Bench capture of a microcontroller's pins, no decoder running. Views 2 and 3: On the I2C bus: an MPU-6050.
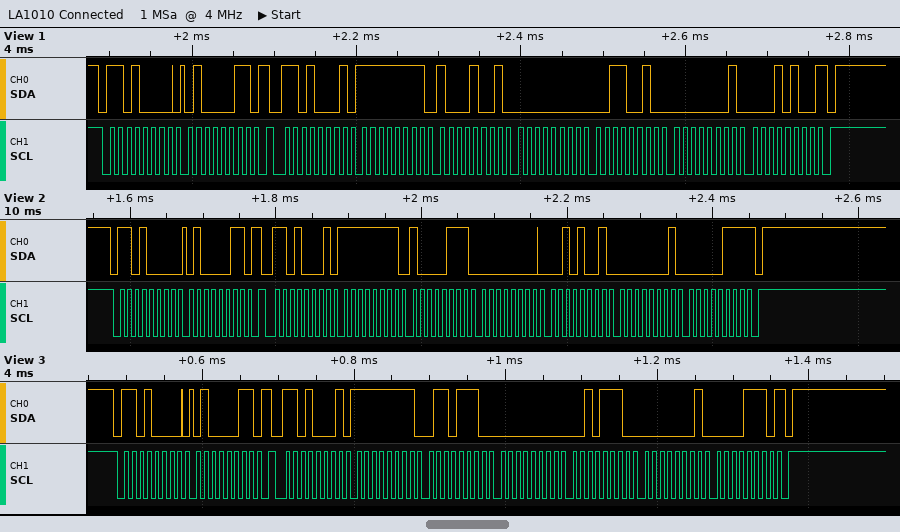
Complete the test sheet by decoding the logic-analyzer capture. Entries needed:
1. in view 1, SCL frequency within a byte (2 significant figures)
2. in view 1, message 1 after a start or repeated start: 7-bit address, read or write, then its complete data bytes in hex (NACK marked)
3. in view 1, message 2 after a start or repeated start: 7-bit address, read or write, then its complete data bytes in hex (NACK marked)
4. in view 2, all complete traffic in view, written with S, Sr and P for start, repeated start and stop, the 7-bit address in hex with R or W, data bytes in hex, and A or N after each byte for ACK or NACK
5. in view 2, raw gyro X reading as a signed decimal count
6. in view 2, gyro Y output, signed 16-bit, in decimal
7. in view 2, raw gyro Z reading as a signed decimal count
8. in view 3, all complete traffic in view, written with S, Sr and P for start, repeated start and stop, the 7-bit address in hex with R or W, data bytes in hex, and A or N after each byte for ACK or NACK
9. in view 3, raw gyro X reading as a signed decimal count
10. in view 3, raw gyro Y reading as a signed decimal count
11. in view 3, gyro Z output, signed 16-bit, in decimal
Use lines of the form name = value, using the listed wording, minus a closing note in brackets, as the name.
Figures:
in view 1, SCL frequency within a byte = 100 kHz
in view 1, message 1 after a start or repeated start: 7-bit address, read or write, then its complete data bytes in hex = 0x68 write: 43
in view 1, message 2 after a start or repeated start: 7-bit address, read or write, then its complete data bytes in hex = 0x68 read: FF 89 00 32 01 14 NACK
in view 2, all complete traffic in view, written with S, Sr and P for start, repeated start and stop, the 7-bit address in hex with R or W, data bytes in hex, and A or N after each byte for ACK or NACK = S 68W A 43 A Sr 68R A FF A 87 A 00 A 29 A 01 A 07 N P
in view 2, raw gyro X reading as a signed decimal count = -121
in view 2, gyro Y output, signed 16-bit, in decimal = 41
in view 2, raw gyro Z reading as a signed decimal count = 263
in view 3, all complete traffic in view, written with S, Sr and P for start, repeated start and stop, the 7-bit address in hex with R or W, data bytes in hex, and A or N after each byte for ACK or NACK = S 68W A 43 A Sr 68R A FF A 6E A 00 A 2E A 01 A 0E N P
in view 3, raw gyro X reading as a signed decimal count = -146
in view 3, raw gyro Y reading as a signed decimal count = 46
in view 3, gyro Z output, signed 16-bit, in decimal = 270
